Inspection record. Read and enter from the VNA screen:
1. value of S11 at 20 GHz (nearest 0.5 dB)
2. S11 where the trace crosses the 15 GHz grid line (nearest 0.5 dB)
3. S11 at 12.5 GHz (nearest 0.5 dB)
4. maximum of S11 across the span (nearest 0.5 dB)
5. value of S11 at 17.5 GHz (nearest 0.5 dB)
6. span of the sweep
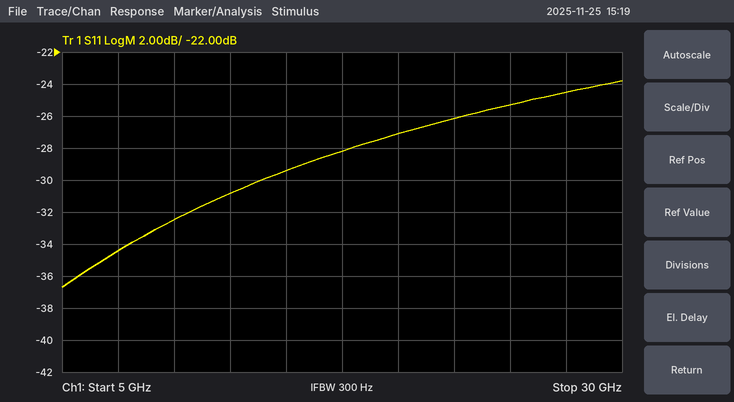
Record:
-27.0 dB
-29.5 dB
-31.0 dB
-24.0 dB
-28.0 dB
25 GHz
